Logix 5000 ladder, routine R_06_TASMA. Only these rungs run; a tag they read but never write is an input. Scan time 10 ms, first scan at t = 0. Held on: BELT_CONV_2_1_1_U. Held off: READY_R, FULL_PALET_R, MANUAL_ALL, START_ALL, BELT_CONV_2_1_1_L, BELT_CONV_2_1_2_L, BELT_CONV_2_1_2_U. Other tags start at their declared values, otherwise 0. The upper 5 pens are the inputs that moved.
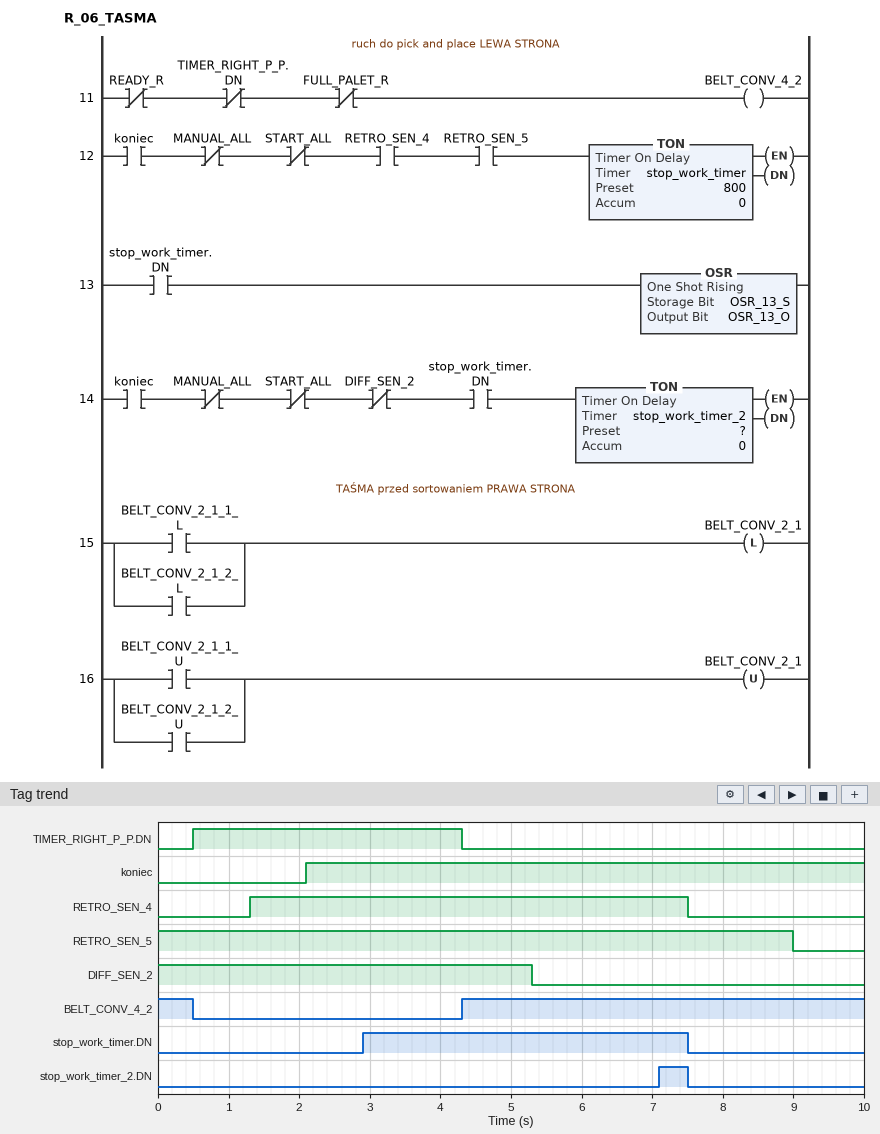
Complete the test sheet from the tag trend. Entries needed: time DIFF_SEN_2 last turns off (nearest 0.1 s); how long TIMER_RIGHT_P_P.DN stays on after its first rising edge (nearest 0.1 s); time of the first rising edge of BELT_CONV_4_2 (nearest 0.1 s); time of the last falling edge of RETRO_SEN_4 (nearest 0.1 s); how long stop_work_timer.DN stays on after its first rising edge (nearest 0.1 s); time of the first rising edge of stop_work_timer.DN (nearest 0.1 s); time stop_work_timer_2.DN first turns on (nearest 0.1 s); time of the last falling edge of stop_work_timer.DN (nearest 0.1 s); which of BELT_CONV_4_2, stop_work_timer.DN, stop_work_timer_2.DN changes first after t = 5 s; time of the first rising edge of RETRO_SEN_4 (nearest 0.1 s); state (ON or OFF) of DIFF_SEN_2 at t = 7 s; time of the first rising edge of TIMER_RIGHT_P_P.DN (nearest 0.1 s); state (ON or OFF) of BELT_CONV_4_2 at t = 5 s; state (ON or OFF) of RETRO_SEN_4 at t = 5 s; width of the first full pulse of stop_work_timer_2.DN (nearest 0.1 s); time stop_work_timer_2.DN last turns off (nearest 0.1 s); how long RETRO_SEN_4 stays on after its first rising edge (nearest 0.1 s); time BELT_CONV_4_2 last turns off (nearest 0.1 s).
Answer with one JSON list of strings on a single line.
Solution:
["5.3 s", "3.8 s", "4.3 s", "7.5 s", "4.6 s", "2.9 s", "7.1 s", "7.5 s", "stop_work_timer_2.DN", "1.3 s", "OFF", "0.5 s", "ON", "ON", "0.4 s", "7.5 s", "6.2 s", "0.5 s"]
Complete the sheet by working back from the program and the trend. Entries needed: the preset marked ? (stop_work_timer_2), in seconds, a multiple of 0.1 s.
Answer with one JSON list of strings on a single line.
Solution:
["1.8 s"]
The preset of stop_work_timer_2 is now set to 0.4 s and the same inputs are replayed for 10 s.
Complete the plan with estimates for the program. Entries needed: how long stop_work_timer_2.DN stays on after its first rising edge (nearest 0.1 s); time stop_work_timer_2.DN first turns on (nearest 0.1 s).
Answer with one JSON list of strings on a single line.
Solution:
["1.8 s", "5.7 s"]
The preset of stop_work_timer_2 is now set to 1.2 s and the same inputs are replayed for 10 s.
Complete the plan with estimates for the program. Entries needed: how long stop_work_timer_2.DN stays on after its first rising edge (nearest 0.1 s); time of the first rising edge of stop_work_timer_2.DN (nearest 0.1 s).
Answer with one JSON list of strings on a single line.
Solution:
["1.0 s", "6.5 s"]
